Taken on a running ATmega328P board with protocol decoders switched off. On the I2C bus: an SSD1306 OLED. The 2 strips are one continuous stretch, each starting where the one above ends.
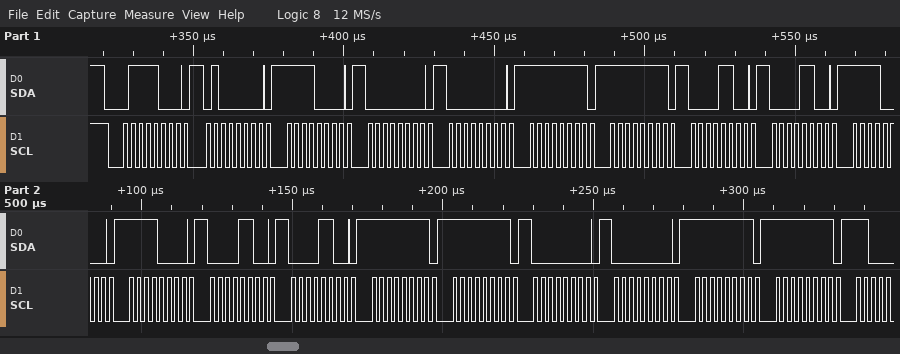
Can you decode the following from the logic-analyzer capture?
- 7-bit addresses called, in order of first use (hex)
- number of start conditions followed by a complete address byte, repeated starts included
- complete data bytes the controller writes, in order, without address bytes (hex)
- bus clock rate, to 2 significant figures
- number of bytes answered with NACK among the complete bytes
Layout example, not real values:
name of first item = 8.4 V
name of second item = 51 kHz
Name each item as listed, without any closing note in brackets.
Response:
7-bit addresses called, in order of first use = 0x3C
number of start conditions followed by a complete address byte, repeated starts included = 1
complete data bytes the controller writes, in order, without address bytes = 40 F0 00 00 FF FF 0C 0C F0 F0 0C 0C FF FF 00 00 FF FF
bus clock rate, to 2 significant figures = 400 kHz
number of bytes answered with NACK among the complete bytes = 0
